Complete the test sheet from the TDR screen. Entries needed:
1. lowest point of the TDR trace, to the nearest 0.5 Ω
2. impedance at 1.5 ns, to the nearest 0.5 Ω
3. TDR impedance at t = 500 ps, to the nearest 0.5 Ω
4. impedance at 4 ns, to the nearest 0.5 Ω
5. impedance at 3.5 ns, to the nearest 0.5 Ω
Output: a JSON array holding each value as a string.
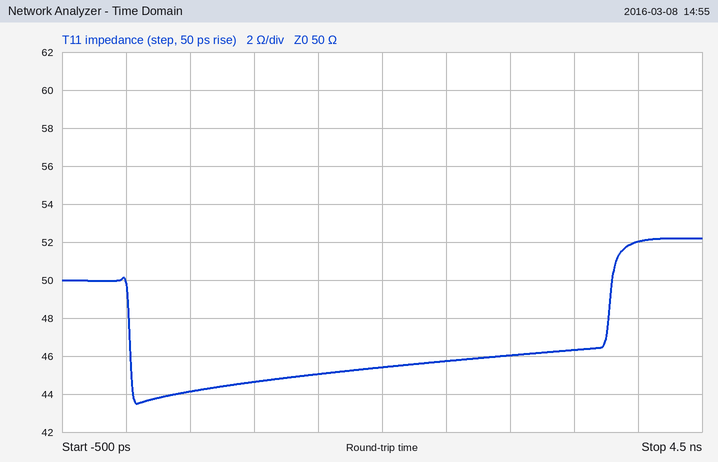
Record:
["43.5 Ω", "45.0 Ω", "44.0 Ω", "52.0 Ω", "46.5 Ω"]
